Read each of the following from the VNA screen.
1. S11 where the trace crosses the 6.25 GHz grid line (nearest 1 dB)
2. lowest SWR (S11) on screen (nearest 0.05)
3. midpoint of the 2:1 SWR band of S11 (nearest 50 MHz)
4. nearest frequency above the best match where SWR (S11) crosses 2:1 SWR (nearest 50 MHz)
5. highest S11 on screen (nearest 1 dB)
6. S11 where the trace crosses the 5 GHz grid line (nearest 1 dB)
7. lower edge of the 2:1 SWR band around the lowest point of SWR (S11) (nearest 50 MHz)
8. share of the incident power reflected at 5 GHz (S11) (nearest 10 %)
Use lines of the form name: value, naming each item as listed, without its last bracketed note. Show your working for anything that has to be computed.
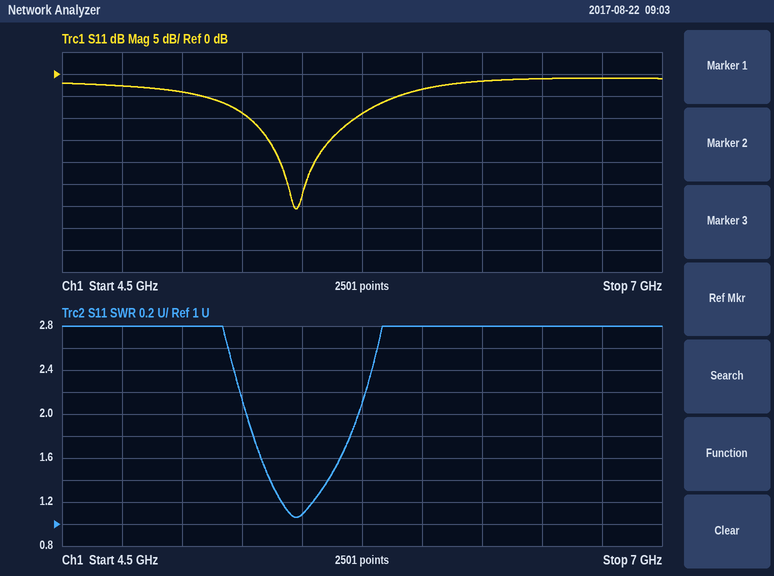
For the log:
S11 where the trace crosses the 6.25 GHz grid line: -2 dB
lowest SWR (S11) on screen: 1.05
midpoint of the 2:1 SWR band of S11: 5.50 GHz
nearest frequency above the best match where SWR (S11) crosses 2:1 SWR: 5.75 GHz
highest S11 on screen: -1 dB
S11 where the trace crosses the 5 GHz grid line: -4 dB
lower edge of the 2:1 SWR band around the lowest point of SWR (S11): 5.25 GHz
share of the incident power reflected at 5 GHz (S11): 10^(-4/10) ≈ 40 %
